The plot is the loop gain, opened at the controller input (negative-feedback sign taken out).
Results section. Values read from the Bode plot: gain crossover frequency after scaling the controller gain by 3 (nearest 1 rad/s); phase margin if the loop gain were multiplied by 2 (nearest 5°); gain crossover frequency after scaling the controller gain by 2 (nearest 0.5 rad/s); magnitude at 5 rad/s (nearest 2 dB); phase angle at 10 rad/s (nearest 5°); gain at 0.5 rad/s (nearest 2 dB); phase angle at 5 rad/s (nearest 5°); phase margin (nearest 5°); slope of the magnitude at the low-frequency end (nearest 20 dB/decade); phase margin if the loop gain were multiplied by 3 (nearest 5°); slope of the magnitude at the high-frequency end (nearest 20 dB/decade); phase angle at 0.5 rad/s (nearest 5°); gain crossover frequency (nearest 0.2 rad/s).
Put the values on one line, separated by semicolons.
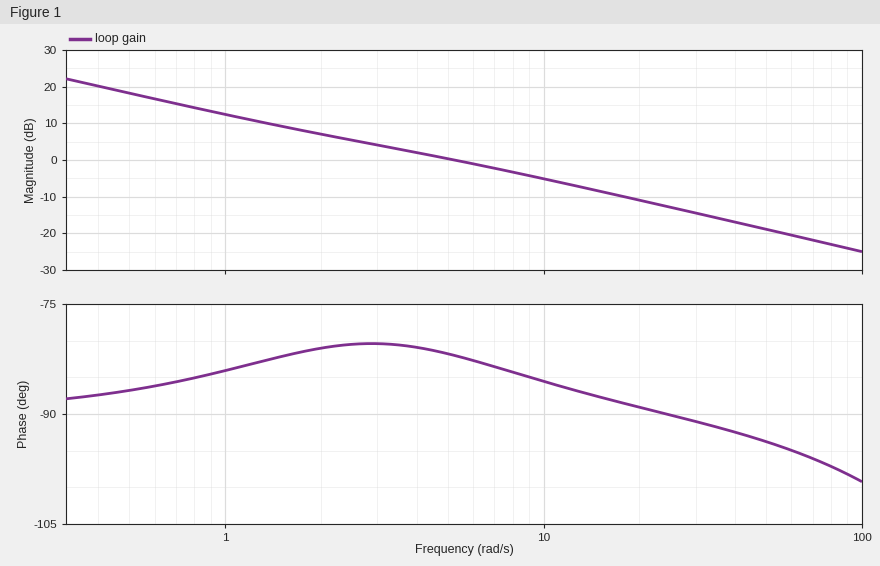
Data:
17 rad/s; 95°; 11.0 rad/s; 0 dB; -85°; 18 dB; -80°; 100°; -20 dB/decade; 90°; -20 dB/decade; -85°; 5.2 rad/s
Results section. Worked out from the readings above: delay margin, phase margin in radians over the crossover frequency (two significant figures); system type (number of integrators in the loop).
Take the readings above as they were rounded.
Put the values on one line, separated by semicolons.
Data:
0.34 s; 1
